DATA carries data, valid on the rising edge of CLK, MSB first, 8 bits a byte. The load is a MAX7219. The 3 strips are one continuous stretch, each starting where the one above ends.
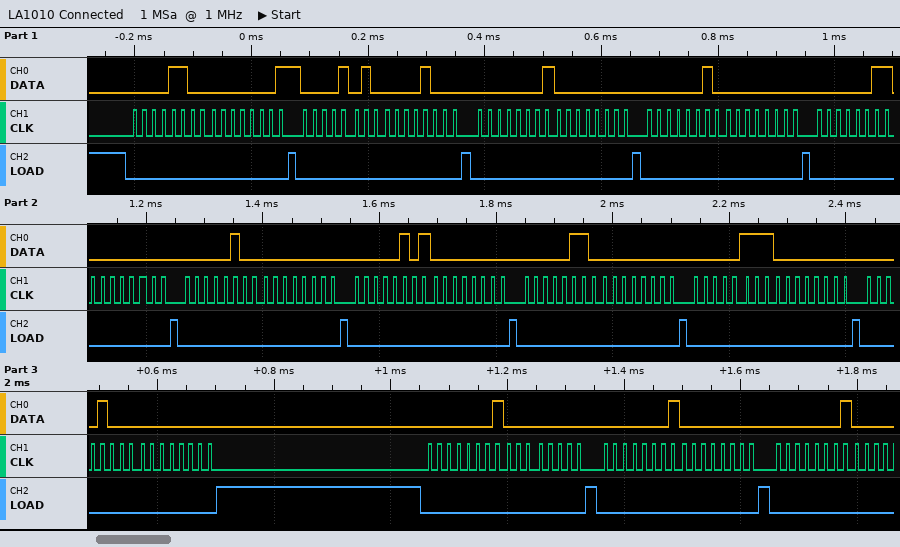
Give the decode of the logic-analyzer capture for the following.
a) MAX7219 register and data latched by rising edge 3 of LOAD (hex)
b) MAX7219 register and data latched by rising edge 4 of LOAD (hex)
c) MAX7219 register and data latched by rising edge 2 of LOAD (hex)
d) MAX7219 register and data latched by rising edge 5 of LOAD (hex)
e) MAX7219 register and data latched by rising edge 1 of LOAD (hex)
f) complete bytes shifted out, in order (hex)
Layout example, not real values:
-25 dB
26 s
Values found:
register 0x1, data 0x00
register 0x2, data 0x00
register 0xA, data 0x08
register 0x3, data 0x00
register 0xC, data 0x01
0C 01 0A 08 01 00 02 00 03 00 04 00 05 00 06 00 07 00 08 00 01 00 01 00 01
